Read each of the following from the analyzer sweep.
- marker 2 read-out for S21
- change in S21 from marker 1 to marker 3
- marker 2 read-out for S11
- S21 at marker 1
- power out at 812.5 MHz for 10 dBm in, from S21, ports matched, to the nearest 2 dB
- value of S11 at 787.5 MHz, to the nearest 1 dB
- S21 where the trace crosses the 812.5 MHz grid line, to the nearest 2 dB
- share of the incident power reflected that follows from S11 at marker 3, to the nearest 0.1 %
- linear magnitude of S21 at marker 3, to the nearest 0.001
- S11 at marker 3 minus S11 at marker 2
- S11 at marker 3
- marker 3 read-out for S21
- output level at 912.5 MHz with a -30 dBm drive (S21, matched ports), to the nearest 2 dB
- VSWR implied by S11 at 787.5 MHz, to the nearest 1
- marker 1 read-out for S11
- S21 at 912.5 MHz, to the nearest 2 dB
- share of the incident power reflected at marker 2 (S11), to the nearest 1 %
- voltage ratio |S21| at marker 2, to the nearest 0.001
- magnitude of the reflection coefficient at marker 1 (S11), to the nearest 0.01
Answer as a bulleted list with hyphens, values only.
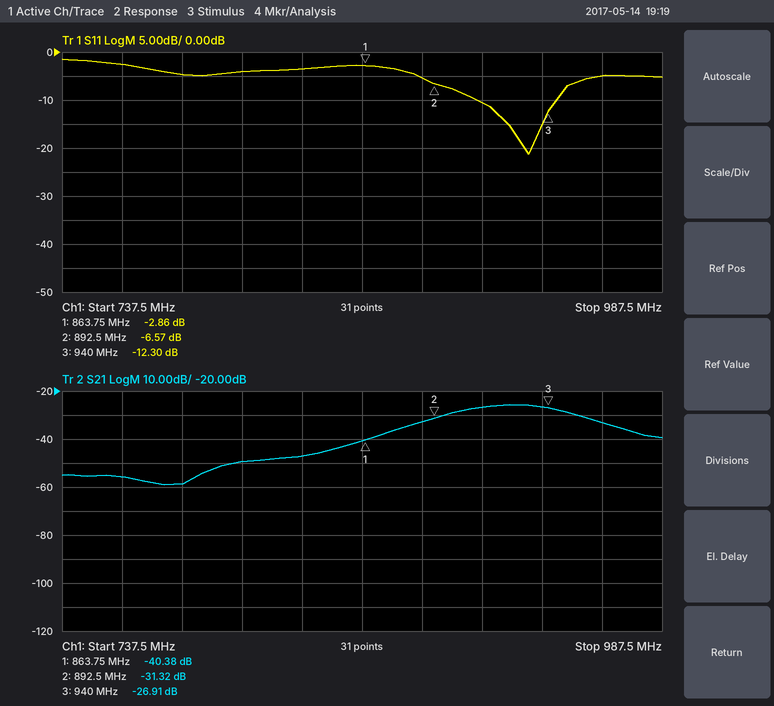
- -31.32 dB
- 13.47 dB
- -6.57 dB
- -40.38 dB
- -40 dBm
- -5 dB
- -50 dB
- 5.9 %
- 0.045
- -5.73 dB
- -12.30 dB
- -26.91 dB
- -56 dBm
- 4
- -2.86 dB
- -26 dB
- 22 %
- 0.027
- 0.72
